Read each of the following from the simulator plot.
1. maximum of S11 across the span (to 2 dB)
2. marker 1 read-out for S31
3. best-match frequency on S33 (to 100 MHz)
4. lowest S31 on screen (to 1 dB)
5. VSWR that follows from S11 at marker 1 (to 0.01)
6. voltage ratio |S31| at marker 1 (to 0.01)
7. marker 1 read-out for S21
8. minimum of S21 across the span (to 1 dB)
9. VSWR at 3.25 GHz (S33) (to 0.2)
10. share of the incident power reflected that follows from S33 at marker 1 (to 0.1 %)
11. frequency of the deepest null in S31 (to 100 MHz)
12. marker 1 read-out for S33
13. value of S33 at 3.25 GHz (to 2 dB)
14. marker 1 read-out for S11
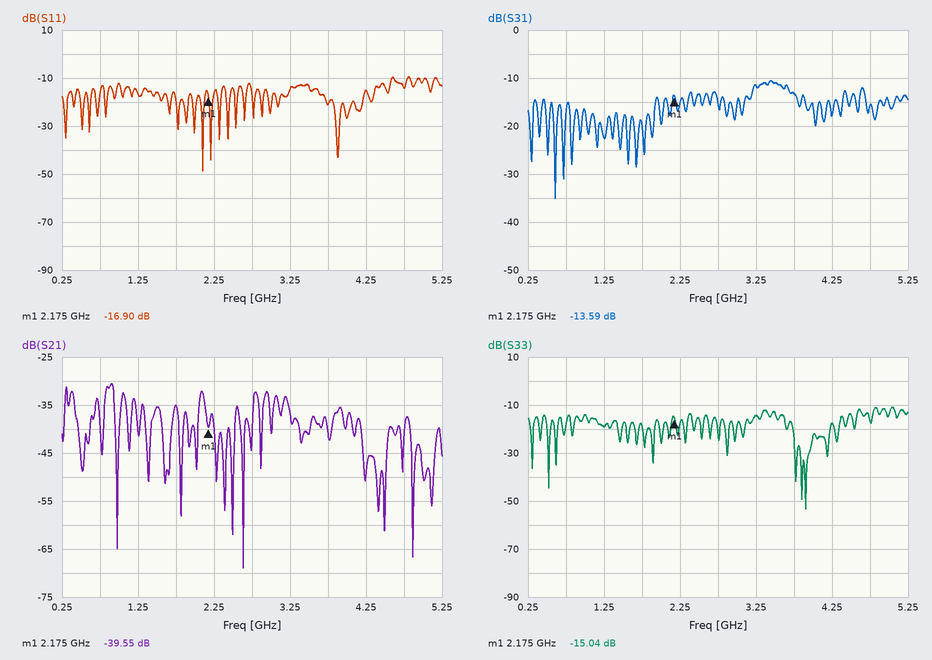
-10 dB
-13.59 dB
3.9 GHz
-35 dB
1.33
0.21
-39.55 dB
-69 dB
1.4
3.1 %
600 MHz
-15.04 dB
-14 dB
-16.90 dB
